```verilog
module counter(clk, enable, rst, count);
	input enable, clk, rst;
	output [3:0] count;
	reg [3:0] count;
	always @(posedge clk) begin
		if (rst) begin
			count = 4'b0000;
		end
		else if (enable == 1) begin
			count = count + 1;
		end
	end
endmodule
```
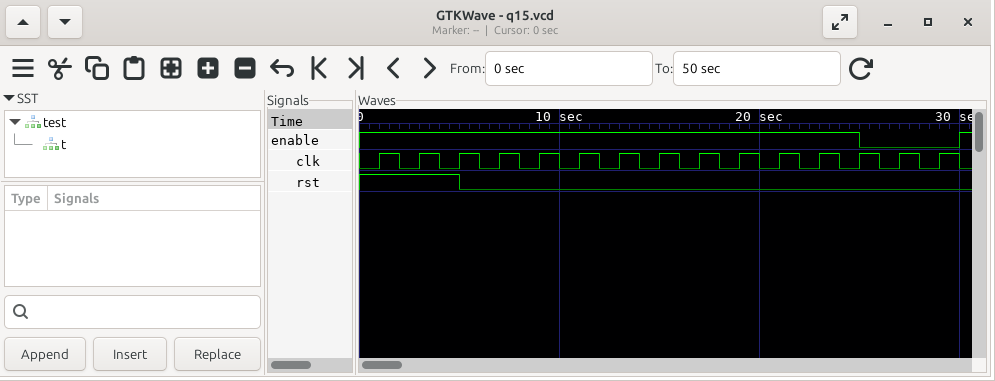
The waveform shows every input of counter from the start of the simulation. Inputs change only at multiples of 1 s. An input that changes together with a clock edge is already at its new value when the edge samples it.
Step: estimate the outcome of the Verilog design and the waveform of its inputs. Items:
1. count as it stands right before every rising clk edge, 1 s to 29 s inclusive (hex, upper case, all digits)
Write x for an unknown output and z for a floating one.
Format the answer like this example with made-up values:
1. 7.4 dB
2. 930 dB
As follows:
1. x, 0, 0, 1, 2, 3, 4, 5, 6, 7, 8, 9, A, A, A
